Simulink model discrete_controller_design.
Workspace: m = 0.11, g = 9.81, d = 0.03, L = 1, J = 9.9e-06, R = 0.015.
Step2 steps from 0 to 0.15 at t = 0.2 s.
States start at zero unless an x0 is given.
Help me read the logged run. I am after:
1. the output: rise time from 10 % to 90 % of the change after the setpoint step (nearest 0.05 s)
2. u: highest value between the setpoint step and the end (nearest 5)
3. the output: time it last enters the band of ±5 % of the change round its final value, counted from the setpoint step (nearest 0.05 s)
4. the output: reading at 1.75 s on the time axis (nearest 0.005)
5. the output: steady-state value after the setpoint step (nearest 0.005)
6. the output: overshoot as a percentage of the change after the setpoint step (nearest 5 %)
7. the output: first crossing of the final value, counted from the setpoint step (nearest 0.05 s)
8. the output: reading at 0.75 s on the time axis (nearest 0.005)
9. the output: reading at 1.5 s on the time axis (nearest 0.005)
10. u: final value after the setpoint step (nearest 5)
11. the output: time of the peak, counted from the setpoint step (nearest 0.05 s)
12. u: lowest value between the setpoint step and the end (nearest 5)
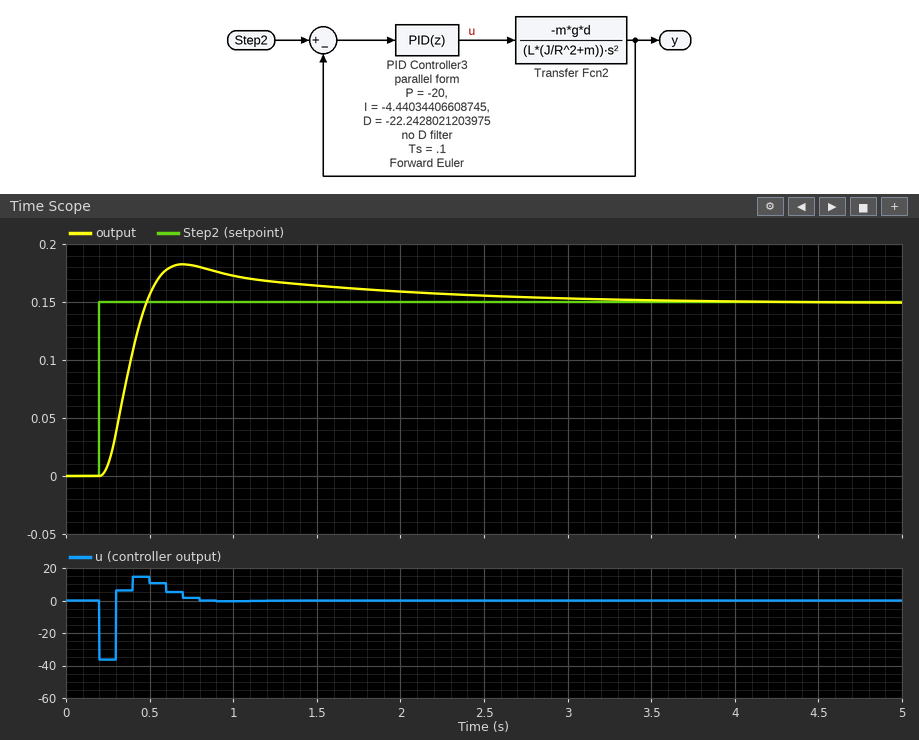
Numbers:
0.20 s
15
2.00 s
0.160
0.150
20 %
0.30 s
0.180
0.165
0
0.50 s
-35
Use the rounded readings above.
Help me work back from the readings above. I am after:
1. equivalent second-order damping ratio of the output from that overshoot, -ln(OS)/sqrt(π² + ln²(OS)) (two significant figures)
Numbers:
0.46
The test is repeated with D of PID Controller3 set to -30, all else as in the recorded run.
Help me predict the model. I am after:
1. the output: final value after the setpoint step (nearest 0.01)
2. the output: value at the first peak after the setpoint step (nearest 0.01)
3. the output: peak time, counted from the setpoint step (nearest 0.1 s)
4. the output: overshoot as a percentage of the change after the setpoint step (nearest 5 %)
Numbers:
0.15
0.19
0.4 s
25 %
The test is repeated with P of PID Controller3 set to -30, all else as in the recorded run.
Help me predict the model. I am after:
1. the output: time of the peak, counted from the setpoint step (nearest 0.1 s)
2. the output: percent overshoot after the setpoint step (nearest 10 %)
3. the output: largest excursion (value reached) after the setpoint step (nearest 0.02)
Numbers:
0.5 s
30 %
0.20
